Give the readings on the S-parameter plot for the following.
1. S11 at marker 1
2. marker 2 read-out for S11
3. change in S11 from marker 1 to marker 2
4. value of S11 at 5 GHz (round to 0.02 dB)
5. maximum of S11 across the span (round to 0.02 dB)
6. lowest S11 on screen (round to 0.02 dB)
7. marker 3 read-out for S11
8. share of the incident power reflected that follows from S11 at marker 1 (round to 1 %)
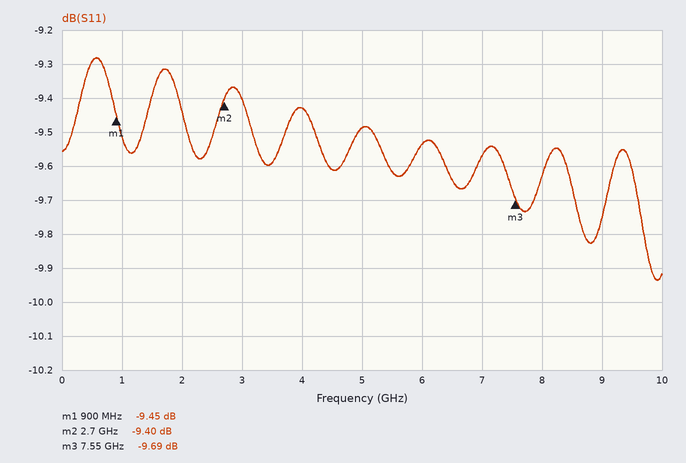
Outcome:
-9.45 dB
-9.40 dB
0.05 dB
-9.48 dB
-9.28 dB
-9.94 dB
-9.69 dB
11 %
